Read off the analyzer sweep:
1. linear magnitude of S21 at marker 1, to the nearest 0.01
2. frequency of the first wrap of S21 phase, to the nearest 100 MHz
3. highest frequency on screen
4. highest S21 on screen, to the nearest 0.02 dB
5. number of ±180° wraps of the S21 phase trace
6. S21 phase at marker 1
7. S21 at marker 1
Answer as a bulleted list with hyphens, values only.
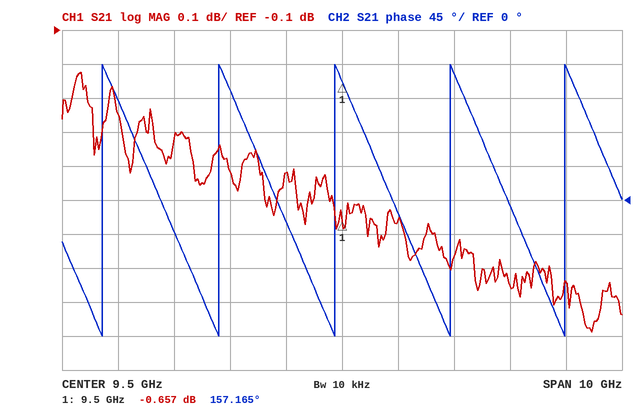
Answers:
- 0.93
- 5.2 GHz
- 14.5 GHz
- -0.22 dB
- 5
- 157.165°
- -0.657 dB
